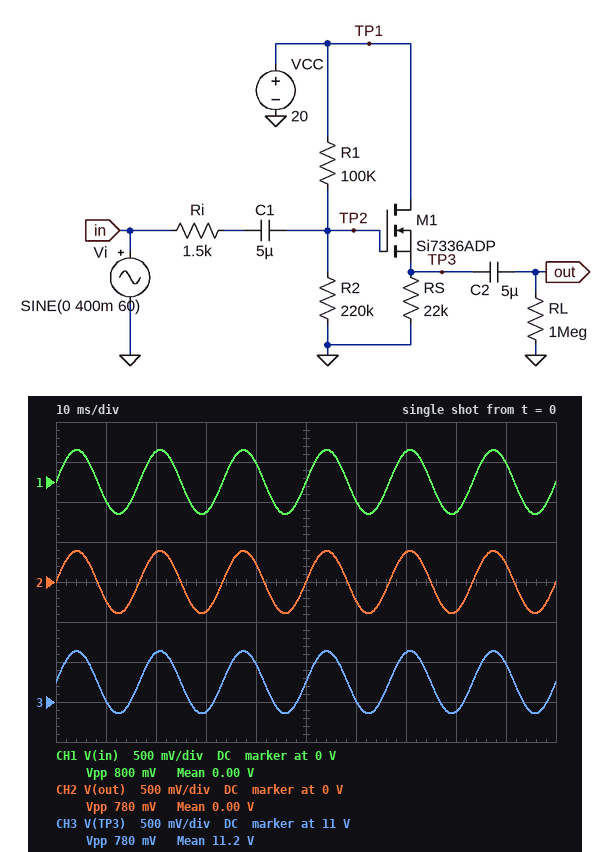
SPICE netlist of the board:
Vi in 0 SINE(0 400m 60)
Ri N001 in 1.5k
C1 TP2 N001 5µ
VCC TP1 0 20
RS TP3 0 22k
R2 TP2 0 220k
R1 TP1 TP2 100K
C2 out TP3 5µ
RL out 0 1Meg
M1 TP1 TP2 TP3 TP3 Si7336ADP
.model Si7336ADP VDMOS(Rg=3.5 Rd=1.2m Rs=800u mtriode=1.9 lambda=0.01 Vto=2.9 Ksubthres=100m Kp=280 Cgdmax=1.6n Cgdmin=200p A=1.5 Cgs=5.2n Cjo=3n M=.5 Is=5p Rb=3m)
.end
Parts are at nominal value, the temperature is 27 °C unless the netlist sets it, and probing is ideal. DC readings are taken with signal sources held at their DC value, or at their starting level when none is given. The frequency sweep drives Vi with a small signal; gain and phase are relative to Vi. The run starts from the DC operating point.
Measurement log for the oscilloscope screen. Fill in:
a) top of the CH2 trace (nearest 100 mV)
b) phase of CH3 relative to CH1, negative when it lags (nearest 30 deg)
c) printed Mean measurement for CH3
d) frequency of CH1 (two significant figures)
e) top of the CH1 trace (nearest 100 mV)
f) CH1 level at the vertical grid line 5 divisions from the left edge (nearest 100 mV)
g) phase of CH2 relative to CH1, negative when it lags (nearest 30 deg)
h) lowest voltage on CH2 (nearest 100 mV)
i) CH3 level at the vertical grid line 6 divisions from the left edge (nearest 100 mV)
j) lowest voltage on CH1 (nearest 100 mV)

400 mV
0 deg
11.2 V
60 Hz
400 mV
0 V
0 deg
-400 mV
11.0 V
-400 mV
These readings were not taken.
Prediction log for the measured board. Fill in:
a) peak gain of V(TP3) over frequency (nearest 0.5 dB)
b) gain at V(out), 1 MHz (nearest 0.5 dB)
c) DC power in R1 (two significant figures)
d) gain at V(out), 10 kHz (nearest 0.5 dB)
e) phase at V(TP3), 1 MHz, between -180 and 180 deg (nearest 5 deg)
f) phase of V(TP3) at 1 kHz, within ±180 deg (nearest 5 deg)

1.0 dB
-20.5 dB
390 µW
0 dB
-95 deg
0 deg
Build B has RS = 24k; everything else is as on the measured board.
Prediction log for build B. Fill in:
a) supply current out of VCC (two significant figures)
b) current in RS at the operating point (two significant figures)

530 µA
470 µA
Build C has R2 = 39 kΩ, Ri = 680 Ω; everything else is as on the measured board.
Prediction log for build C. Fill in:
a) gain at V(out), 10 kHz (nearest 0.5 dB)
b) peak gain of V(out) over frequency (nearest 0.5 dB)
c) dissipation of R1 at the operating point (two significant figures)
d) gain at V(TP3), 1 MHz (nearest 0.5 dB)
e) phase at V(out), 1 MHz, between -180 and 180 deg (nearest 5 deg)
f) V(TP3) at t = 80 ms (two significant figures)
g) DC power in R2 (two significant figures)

-0.5 dB
0 dB
2.1 mW
-12.0 dB
-75 deg
2.8 V
810 µW
